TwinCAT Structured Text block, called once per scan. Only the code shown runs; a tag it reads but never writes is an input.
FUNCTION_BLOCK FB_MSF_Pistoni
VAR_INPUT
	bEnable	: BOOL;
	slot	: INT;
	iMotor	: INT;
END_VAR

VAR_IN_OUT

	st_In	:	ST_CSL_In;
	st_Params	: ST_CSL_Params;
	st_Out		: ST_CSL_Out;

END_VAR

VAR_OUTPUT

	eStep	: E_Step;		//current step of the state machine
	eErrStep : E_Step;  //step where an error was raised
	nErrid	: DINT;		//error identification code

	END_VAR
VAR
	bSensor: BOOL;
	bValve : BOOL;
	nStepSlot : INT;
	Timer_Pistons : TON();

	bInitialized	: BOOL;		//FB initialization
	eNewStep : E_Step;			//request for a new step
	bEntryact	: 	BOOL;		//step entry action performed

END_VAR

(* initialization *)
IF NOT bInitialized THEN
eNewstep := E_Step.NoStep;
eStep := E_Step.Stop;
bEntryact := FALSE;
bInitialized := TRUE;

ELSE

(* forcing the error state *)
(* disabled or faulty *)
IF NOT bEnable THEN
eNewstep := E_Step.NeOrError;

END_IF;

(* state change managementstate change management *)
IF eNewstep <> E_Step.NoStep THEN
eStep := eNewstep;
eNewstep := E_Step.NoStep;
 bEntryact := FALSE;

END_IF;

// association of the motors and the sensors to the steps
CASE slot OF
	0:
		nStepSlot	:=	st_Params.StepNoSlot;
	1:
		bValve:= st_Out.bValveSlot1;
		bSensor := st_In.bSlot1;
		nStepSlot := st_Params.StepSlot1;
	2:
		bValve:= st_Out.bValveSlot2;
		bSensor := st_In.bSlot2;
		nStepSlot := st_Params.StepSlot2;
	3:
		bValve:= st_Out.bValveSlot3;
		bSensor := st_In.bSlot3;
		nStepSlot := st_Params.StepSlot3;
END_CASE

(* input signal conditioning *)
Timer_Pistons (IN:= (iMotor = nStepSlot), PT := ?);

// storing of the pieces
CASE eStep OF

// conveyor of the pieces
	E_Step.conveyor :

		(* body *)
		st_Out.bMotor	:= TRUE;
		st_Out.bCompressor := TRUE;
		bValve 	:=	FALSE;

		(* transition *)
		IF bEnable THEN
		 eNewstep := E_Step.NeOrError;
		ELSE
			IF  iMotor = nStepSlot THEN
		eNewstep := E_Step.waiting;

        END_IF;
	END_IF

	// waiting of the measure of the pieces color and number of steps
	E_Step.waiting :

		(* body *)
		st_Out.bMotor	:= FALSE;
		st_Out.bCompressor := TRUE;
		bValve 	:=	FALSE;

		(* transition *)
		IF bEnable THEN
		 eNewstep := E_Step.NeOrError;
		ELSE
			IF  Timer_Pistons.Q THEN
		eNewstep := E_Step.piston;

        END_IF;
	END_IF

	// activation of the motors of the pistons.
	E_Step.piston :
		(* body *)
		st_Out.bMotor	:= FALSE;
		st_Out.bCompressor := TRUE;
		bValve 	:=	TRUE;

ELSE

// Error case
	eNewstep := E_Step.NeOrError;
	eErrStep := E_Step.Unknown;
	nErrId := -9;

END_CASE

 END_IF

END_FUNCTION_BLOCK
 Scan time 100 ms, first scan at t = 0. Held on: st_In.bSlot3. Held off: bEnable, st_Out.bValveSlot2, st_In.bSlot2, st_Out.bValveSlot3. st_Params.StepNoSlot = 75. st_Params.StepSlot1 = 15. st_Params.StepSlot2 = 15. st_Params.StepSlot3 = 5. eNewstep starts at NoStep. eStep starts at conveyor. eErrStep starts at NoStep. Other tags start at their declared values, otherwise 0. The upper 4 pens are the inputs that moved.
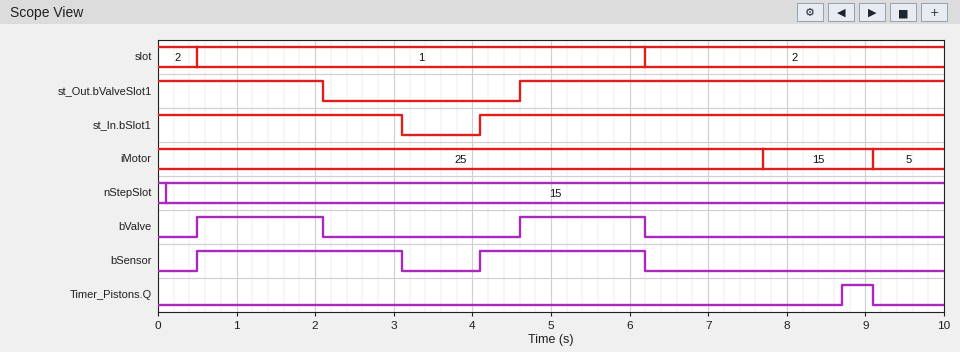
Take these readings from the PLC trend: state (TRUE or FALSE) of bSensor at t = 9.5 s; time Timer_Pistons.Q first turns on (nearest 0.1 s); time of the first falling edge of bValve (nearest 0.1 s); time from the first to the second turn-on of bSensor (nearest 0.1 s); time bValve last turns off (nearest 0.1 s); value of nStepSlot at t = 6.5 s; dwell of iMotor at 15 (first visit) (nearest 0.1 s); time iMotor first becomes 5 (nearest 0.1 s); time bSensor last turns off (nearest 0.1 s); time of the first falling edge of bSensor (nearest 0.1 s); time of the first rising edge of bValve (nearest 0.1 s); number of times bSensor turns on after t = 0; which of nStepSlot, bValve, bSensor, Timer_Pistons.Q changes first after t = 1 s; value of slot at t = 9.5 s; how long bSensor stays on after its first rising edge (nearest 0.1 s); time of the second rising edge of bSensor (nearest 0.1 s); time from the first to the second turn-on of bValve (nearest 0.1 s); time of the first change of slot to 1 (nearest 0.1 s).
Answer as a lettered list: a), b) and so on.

a) FALSE
b) 8.7 s
c) 2.1 s
d) 3.6 s
e) 6.2 s
f) 15
g) 1.4 s
h) 9.1 s
i) 6.2 s
j) 3.1 s
k) 0.5 s
l) 2
m) bValve
n) 2
o) 2.6 s
p) 4.1 s
q) 4.1 s
r) 0.5 s
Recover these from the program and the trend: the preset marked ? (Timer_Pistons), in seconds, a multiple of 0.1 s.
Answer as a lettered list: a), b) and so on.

a) 1.0 s
